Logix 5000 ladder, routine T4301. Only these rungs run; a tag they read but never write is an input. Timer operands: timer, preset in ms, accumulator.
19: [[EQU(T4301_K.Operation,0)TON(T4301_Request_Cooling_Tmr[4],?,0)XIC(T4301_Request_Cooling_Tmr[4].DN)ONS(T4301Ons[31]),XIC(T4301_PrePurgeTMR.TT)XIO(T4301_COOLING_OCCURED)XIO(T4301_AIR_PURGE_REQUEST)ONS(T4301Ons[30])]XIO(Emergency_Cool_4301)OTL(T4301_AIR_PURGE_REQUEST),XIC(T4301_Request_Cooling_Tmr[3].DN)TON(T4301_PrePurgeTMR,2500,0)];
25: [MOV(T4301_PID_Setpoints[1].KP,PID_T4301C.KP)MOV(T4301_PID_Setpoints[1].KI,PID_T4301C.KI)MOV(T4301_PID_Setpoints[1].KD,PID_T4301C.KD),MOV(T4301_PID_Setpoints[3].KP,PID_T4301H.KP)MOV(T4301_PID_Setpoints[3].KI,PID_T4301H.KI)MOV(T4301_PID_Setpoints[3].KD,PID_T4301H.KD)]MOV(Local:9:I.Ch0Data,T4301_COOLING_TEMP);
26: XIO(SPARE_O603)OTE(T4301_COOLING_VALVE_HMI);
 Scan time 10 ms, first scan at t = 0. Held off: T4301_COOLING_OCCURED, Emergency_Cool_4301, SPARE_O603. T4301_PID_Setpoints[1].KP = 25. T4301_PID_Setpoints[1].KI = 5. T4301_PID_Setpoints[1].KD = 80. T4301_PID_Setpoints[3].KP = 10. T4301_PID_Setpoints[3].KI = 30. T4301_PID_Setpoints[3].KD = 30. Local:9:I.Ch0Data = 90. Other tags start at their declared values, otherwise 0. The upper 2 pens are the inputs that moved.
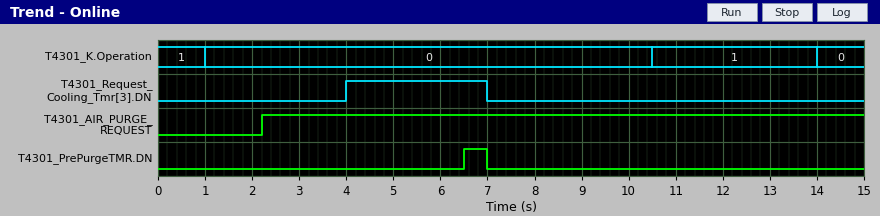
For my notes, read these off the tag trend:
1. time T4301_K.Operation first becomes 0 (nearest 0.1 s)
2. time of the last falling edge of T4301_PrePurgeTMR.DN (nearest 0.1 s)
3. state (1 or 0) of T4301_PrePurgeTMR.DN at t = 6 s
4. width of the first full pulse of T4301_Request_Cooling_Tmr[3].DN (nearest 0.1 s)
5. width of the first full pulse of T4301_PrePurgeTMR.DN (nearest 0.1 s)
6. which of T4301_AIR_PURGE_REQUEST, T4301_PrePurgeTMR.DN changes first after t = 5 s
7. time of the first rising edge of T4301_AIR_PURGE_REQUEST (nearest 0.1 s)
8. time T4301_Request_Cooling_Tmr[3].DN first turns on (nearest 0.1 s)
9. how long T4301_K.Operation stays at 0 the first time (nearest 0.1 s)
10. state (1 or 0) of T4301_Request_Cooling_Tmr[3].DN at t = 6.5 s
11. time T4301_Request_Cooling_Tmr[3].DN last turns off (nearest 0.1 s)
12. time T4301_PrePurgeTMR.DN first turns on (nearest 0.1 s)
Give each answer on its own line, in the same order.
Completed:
1.0 s
7.0 s
0
3.0 s
0.5 s
T4301_PrePurgeTMR.DN
2.2 s
4.0 s
9.5 s
1
7.0 s
6.5 s
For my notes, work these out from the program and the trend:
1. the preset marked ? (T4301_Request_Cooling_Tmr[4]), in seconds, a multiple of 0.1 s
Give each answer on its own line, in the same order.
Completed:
1.2 s
